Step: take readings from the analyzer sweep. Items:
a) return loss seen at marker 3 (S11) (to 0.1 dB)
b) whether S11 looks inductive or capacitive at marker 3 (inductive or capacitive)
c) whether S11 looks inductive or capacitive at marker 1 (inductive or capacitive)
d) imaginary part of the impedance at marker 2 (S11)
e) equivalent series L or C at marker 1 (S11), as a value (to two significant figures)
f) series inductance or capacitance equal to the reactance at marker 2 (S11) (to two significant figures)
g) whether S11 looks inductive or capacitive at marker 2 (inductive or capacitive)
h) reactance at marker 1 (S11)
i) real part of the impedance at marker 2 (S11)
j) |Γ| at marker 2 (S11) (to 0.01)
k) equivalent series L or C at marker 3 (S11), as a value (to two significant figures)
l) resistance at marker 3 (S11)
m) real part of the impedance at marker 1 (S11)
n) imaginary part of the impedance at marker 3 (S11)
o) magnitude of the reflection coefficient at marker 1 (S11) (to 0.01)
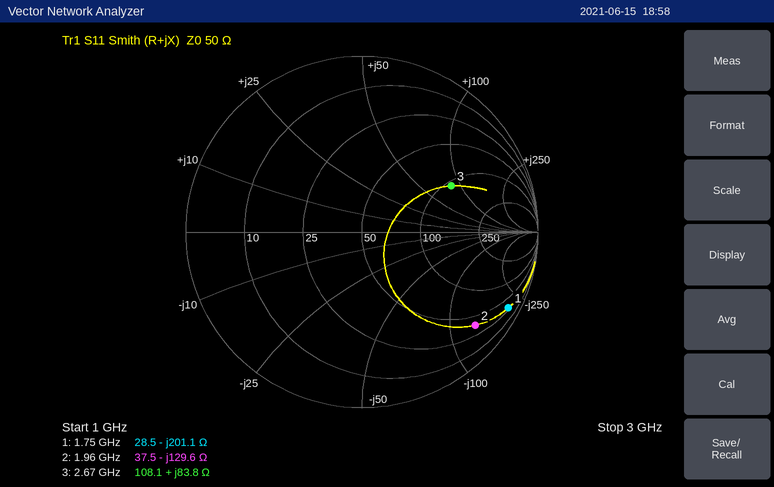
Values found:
4.9 dB
inductive
capacitive
-129.6 Ω
450 fF
630 fF
capacitive
-201.1 Ω
37.5 Ω
0.83
5.0 nH
108.1 Ω
28.5 Ω
+83.8 Ω
0.94
